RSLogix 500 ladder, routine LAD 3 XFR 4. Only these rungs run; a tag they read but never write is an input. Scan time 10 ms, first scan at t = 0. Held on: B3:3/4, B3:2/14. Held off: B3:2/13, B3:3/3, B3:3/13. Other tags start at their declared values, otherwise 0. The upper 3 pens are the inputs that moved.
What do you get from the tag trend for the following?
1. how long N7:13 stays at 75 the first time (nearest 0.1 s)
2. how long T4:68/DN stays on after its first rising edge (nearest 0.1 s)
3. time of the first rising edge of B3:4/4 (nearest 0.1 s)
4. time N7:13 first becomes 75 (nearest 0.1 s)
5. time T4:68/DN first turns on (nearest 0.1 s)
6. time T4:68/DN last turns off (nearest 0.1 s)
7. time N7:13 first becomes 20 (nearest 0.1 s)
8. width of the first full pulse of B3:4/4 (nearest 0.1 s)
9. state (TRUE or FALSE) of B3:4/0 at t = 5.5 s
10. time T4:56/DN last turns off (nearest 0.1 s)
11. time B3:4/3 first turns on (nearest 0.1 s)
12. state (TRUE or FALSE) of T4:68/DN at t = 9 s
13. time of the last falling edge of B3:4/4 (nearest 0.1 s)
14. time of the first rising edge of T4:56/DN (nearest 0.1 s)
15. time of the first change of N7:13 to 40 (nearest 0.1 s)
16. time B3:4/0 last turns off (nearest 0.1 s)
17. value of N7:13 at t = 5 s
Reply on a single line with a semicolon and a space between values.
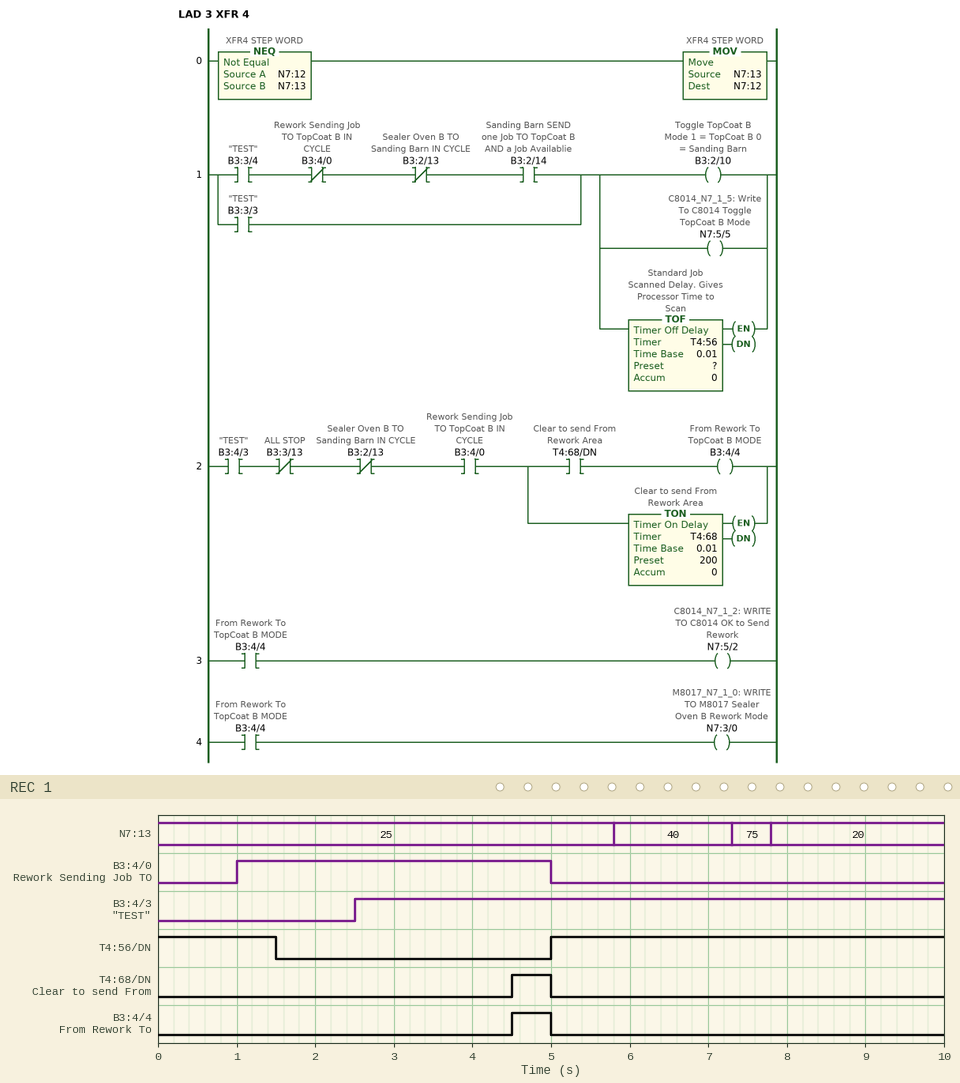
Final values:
0.5 s; 0.5 s; 4.5 s; 7.3 s; 4.5 s; 5.0 s; 7.8 s; 0.5 s; FALSE; 1.5 s; 2.5 s; FALSE; 5.0 s; 5.0 s; 5.8 s; 5.0 s; 25
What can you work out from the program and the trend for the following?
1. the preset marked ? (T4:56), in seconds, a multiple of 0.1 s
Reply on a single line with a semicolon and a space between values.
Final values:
0.5 s
